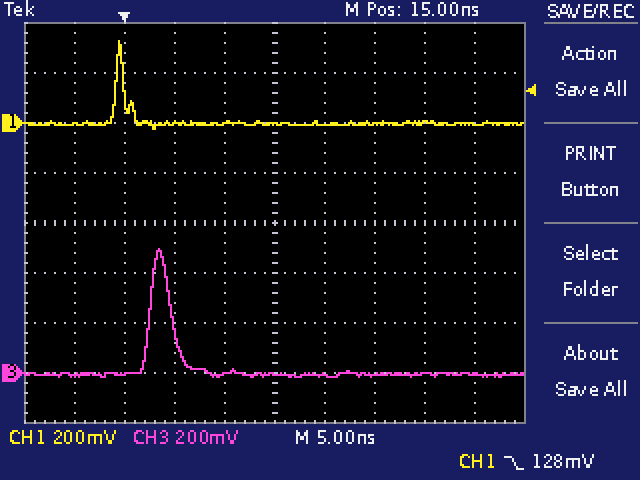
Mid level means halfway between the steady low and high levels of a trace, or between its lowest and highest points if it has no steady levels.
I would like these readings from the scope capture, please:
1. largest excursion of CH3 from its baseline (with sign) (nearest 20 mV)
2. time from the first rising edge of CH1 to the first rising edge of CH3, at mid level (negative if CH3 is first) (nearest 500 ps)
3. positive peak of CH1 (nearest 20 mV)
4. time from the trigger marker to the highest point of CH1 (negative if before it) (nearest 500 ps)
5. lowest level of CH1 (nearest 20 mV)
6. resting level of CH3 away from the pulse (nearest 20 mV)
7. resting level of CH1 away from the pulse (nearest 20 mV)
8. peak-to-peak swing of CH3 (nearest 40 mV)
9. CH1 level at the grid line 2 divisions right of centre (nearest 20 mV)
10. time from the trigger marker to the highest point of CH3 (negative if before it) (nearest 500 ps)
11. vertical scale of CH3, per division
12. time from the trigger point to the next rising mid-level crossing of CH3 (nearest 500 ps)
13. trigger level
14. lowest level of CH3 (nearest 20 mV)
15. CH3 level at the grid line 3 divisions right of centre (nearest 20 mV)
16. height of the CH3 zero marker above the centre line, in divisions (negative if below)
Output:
+500 mV
+3.5 ns
320 mV
-500 ps
-20 mV
0 mV
0 mV
520 mV
0 mV
+3.5 ns
200 mV
2.5 ns
128 mV
-20 mV
0 mV
-3.0 div
